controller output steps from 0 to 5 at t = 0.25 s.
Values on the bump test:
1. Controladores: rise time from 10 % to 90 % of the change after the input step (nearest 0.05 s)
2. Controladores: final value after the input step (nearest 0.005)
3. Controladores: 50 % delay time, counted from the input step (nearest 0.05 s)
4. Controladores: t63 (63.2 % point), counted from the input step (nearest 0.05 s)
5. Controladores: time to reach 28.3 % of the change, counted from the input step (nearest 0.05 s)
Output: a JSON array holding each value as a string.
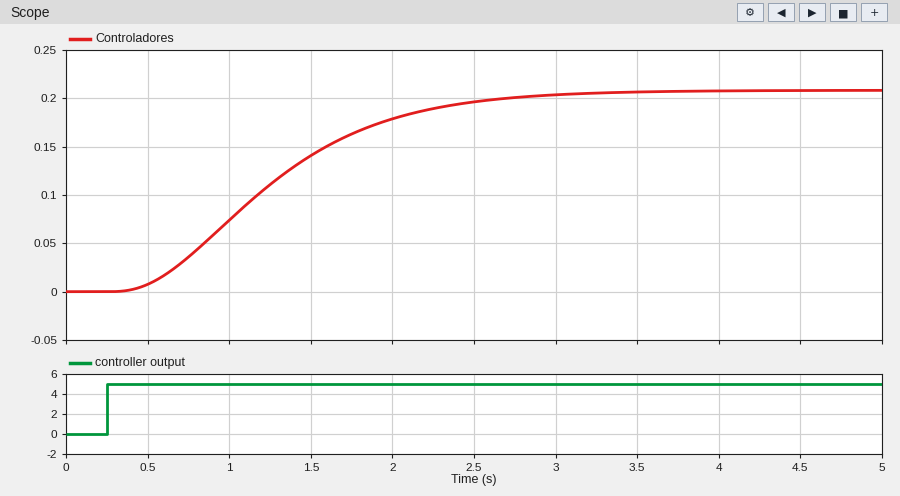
["1.55 s", "0.210", "0.95 s", "1.15 s", "0.65 s"]
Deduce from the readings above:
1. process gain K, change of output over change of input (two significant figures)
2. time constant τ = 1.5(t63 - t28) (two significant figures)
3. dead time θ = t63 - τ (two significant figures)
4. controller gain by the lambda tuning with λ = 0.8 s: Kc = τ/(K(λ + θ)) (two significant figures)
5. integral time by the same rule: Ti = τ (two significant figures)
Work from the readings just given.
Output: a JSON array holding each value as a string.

["0.042", "0.75 s", "0.40 s", "15", "0.75 s"]
